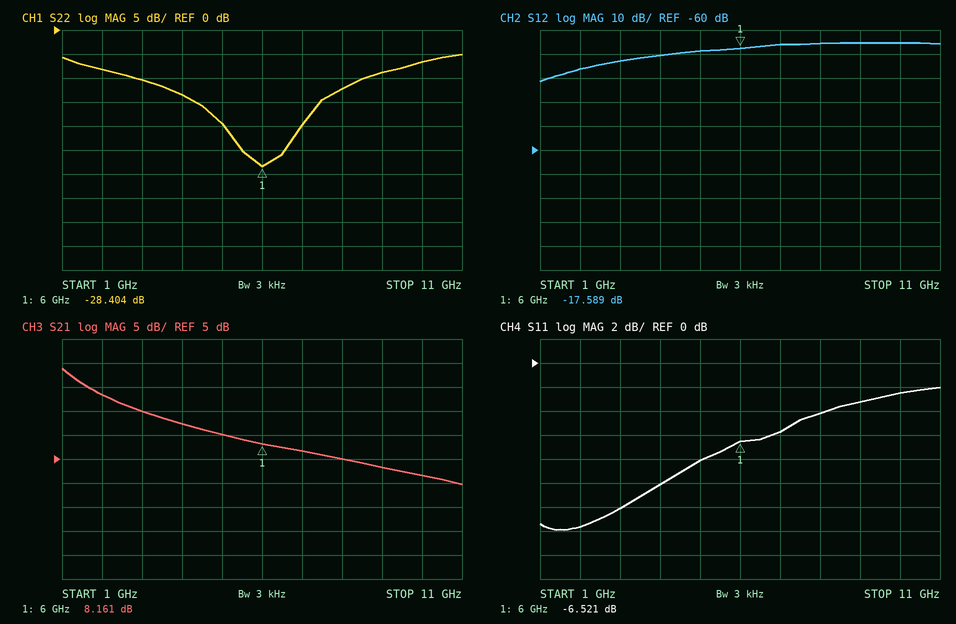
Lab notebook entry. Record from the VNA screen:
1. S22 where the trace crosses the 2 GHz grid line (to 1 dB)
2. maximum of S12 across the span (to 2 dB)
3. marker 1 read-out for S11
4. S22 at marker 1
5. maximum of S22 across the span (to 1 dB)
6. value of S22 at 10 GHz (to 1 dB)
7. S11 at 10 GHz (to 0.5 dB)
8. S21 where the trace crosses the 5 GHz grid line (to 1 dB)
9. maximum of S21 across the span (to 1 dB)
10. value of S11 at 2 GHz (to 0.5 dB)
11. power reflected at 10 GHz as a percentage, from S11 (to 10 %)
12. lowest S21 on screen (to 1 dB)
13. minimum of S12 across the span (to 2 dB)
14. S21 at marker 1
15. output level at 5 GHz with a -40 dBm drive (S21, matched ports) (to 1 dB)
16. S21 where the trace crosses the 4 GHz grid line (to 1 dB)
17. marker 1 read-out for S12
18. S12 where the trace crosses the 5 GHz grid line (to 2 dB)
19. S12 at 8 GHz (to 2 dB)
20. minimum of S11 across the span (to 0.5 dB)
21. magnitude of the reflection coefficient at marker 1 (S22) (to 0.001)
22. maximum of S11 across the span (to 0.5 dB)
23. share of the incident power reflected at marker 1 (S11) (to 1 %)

-8 dB
-16 dB
-6.521 dB
-28.404 dB
-5 dB
-7 dB
-2.5 dB
10 dB
24 dB
-13.5 dB
60 %
0 dB
-32 dB
8.161 dB
-30 dBm
12 dB
-17.589 dB
-18 dB
-16 dB
-14.0 dB
0.038
-2.0 dB
22 %
